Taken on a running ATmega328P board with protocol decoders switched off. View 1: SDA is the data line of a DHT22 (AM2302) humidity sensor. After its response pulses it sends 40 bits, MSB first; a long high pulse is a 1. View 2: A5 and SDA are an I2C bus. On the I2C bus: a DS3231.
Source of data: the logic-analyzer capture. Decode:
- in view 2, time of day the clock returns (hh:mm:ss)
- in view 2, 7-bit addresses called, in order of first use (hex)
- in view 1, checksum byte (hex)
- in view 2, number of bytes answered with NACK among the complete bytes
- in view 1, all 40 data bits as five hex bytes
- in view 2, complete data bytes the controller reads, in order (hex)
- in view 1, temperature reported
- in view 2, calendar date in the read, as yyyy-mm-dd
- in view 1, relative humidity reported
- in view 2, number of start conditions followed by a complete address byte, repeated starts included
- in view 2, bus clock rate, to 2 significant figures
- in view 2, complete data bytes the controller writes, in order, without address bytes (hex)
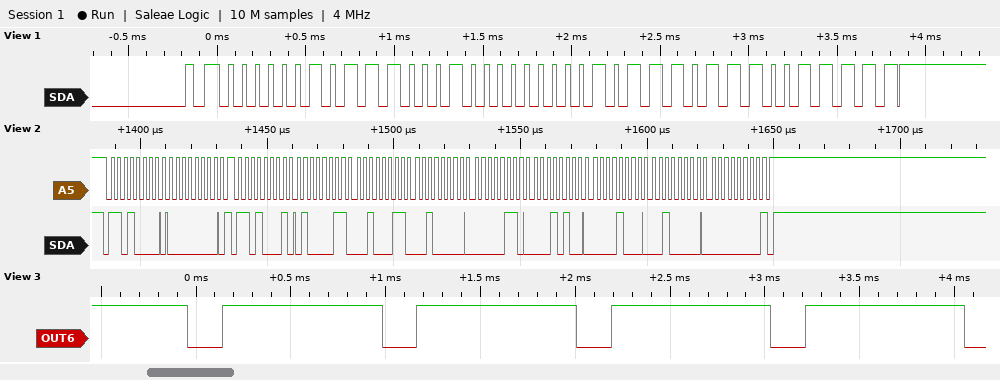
20:23:43
0x68
0x9F
1
02 E2 00 BB 9F
43 23 20 06 14 08 20 00
18.7 °C
2020-08-14
73.8 %
2
400 kHz
00
